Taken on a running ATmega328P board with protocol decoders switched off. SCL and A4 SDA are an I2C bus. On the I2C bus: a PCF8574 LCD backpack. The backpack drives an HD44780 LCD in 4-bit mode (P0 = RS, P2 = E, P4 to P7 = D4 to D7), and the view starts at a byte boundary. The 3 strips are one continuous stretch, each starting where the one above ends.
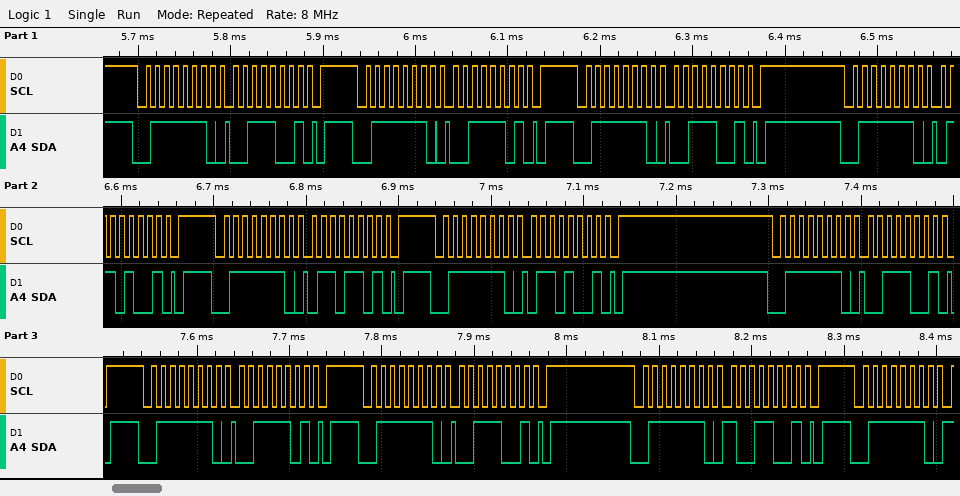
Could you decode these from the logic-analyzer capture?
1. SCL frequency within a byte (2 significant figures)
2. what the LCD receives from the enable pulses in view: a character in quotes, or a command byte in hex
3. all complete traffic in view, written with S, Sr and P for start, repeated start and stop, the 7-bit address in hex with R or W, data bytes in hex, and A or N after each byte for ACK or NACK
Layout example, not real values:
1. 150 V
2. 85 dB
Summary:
1. 100 kHz
2. '6'
3. S 3FW A 39 A P S 3FW A 3D A P S 3FW A 39 A P S 3FW A 69 A P S 3FW A 6D A P S 3FW A 69 A P S 3FW A 39 A P S 3FW A 3D A P S 3FW A 39 A P S 3FW A 99 A P S 3FW A
